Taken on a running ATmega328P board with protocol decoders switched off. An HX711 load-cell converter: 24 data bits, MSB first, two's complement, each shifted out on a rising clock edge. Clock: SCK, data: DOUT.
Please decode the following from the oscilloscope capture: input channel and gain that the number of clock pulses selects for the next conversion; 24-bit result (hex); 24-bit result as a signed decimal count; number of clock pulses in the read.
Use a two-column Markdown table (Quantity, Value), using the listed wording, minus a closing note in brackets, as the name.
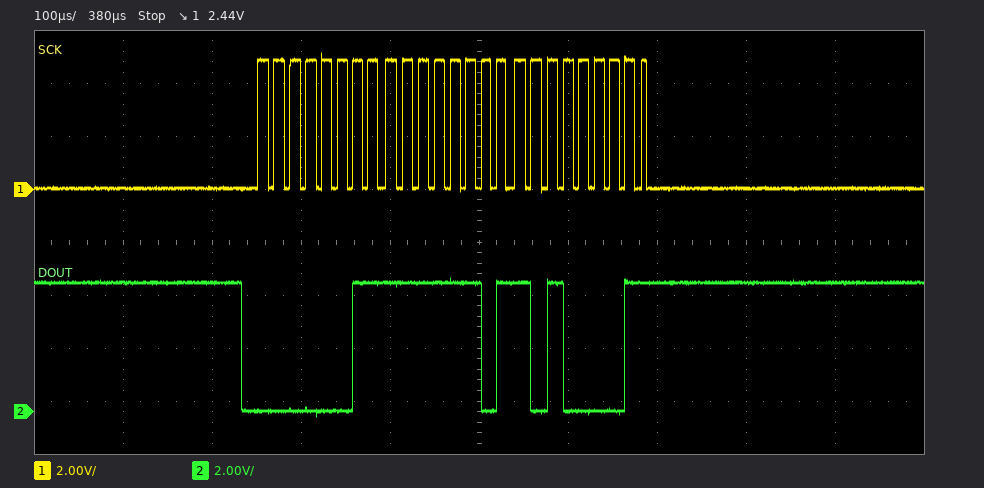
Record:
| Quantity | Value |
|---|---|
| input channel and gain that the number of clock pulses selects for the next conversion | channel A, gain 128 |
| 24-bit result | 0x03FDA1 |
| 24-bit result as a signed decimal count | 261537 |
| number of clock pulses in the read | 25 |
